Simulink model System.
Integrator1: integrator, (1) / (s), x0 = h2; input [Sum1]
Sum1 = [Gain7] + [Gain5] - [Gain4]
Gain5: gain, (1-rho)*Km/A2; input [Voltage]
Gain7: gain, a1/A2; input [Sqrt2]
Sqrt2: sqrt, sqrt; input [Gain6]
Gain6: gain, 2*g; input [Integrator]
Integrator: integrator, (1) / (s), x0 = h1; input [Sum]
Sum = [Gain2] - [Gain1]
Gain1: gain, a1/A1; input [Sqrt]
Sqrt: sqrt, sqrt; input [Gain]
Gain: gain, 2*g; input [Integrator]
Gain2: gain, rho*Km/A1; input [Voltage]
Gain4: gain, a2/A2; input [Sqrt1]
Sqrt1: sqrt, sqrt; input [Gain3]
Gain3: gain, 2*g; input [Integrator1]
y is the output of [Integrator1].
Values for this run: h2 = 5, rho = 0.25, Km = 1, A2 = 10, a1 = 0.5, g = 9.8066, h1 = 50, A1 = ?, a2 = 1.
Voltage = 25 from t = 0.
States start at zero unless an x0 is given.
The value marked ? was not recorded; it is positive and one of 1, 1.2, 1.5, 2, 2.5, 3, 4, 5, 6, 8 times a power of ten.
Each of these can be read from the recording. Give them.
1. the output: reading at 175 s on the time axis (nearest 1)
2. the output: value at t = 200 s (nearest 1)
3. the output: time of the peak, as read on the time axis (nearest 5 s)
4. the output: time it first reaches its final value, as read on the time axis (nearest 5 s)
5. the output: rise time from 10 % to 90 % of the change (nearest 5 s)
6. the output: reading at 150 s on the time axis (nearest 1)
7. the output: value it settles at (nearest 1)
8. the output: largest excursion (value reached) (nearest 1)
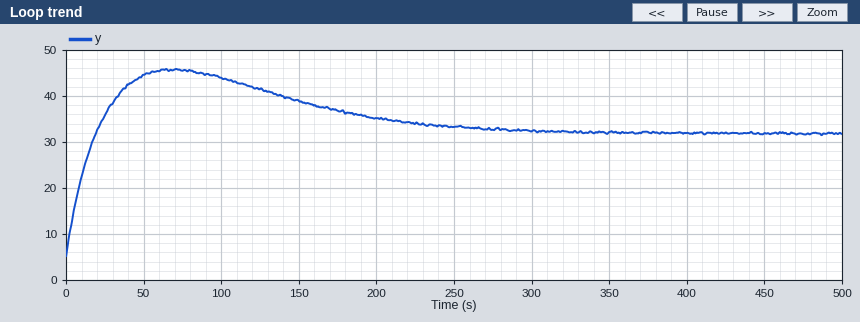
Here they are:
37
35
70 s
20 s
15 s
39
32
46
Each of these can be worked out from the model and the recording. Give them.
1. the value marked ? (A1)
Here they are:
20
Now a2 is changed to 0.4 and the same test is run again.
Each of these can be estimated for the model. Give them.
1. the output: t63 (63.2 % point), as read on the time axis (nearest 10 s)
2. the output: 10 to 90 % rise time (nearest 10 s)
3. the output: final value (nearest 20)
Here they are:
70 s
160 s
200
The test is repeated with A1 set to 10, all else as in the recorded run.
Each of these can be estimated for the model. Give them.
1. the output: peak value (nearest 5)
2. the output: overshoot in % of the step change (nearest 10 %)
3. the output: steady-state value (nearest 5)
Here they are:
40
30 %
30
